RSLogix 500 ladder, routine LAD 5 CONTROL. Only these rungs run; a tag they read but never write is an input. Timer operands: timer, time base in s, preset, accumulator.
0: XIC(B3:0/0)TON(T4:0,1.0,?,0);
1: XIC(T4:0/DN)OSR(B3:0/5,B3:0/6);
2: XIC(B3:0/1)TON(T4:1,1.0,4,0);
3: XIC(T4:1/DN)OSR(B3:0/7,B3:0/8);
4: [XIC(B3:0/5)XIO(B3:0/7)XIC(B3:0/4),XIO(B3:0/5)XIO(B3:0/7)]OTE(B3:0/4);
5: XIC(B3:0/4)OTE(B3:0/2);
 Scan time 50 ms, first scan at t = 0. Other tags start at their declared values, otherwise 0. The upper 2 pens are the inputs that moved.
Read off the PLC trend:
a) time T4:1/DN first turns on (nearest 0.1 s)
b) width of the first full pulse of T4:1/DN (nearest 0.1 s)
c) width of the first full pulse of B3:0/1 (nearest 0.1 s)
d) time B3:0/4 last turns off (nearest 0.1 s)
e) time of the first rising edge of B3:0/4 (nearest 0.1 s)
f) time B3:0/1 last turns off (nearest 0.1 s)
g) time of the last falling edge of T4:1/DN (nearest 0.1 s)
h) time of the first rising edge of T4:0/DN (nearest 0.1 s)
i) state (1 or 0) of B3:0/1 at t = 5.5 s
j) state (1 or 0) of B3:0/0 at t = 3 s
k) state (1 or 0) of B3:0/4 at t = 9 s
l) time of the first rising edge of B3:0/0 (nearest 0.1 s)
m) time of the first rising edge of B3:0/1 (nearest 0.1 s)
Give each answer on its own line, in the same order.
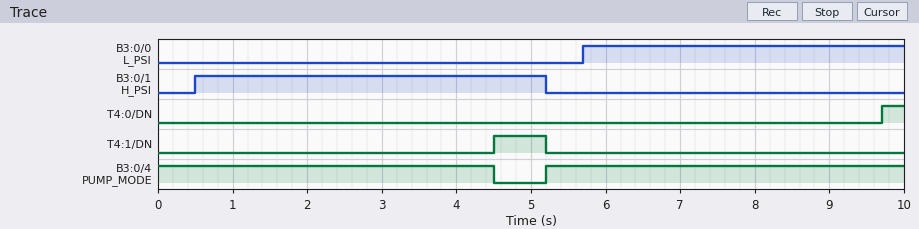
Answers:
4.5 s
0.7 s
4.7 s
4.5 s
5.2 s
5.2 s
5.2 s
9.7 s
0
0
1
5.7 s
0.5 s
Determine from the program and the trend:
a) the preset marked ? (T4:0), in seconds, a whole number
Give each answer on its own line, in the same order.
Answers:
4 s
